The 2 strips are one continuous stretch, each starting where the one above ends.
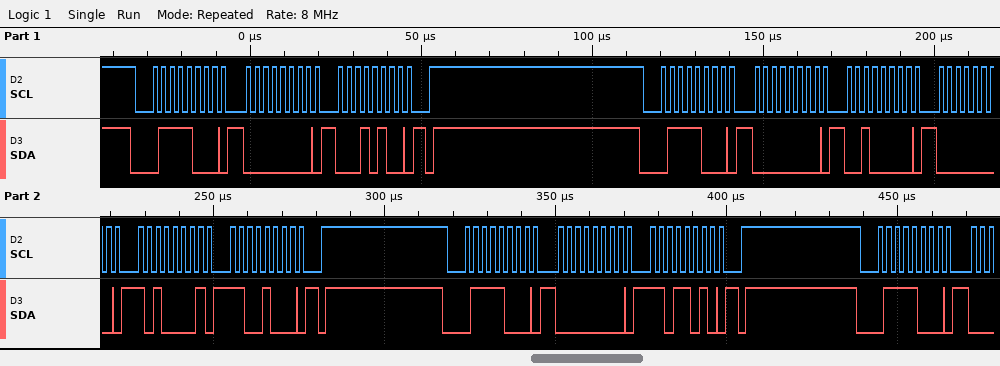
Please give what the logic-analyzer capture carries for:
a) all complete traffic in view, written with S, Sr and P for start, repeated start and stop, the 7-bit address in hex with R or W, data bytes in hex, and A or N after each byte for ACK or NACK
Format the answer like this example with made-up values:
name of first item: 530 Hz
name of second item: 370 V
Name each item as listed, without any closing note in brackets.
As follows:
all complete traffic in view, written with S, Sr and P for start, repeated start and stop, the 7-bit address in hex with R or W, data bytes in hex, and A or N after each byte for ACK or NACK: S 3CW A 00 A 14 A P S 3CW A 00 A 20 A 00 A A1 A C8 A P S 3CW A 00 A DA A P S 3CW A
